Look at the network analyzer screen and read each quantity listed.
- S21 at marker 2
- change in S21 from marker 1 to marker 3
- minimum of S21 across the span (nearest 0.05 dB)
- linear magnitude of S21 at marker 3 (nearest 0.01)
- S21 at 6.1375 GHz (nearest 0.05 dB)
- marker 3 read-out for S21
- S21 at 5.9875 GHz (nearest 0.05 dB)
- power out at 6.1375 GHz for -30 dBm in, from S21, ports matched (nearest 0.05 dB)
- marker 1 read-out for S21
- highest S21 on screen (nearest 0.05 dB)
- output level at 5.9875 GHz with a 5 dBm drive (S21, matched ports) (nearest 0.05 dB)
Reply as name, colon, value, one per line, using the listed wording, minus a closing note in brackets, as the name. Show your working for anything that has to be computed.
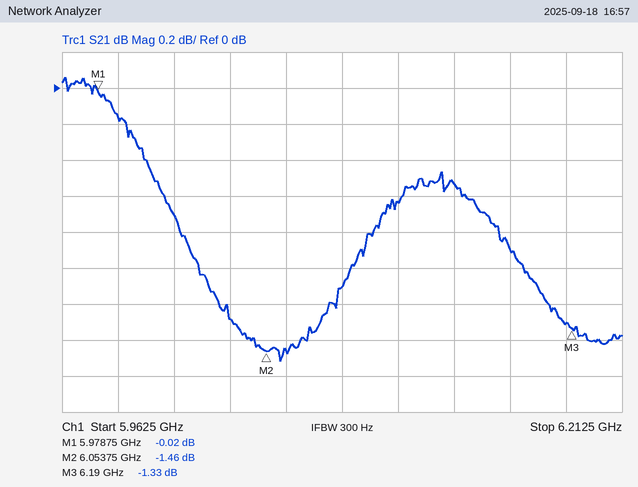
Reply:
S21 at marker 2: -1.46 dB
change in S21 from marker 1 to marker 3: -1.33 − (-0.02) = -1.31 dB
minimum of S21 across the span: -1.50 dB
linear magnitude of S21 at marker 3: 10^(-1.33/20) ≈ 0.86
S21 at 6.1375 GHz: -0.55 dB
marker 3 read-out for S21: -1.33 dB
S21 at 5.9875 GHz: -0.15 dB
power out at 6.1375 GHz for -30 dBm in, from S21, ports matched: -30 dBm + (-0.55 dB) = -30.55 dBm
marker 1 read-out for S21: -0.02 dB
highest S21 on screen: 0.05 dB
output level at 5.9875 GHz with a 5 dBm drive (S21, matched ports): 5 dBm + (-0.15 dB) = 4.85 dBm
